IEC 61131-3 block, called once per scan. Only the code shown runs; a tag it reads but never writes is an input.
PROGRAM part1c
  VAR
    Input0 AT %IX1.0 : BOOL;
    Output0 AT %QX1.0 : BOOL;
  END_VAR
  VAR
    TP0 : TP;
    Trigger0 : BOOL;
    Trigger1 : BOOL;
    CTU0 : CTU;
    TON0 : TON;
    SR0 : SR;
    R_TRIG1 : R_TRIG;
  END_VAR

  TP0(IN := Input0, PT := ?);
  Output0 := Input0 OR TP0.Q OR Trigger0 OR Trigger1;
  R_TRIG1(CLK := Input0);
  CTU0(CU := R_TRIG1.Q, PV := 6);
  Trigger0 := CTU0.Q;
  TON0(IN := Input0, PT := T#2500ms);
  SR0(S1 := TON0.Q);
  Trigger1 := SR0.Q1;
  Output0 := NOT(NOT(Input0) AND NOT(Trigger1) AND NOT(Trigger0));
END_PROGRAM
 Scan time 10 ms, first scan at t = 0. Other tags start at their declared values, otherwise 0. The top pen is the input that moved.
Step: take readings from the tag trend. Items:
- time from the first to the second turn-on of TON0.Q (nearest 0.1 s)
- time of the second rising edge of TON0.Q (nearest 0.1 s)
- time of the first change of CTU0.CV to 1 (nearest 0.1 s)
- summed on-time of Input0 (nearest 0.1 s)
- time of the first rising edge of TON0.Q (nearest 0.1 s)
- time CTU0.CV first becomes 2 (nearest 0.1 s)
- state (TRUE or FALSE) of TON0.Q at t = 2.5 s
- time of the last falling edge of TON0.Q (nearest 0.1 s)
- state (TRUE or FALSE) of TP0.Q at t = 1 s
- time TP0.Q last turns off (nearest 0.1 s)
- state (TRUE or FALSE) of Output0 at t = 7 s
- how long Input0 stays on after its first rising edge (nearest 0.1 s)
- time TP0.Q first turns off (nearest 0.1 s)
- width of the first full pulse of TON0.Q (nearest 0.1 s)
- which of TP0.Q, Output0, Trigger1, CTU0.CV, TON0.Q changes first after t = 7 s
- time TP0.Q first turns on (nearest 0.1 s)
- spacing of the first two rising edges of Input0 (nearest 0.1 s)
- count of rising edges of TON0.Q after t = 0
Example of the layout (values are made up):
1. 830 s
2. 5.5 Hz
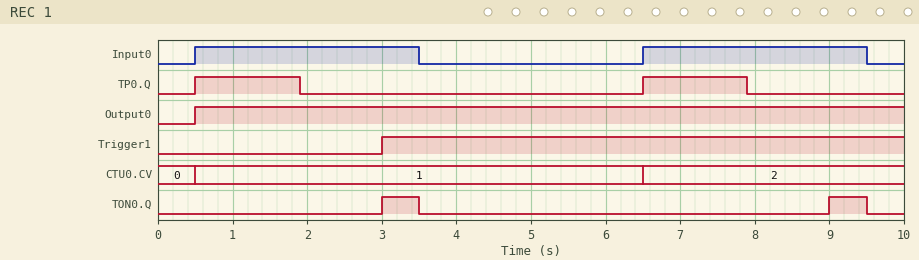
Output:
1. 6.0 s
2. 9.0 s
3. 0.5 s
4. 6.0 s
5. 3.0 s
6. 6.5 s
7. FALSE
8. 9.5 s
9. TRUE
10. 7.9 s
11. TRUE
12. 3.0 s
13. 1.9 s
14. 0.5 s
15. TP0.Q
16. 0.5 s
17. 6.0 s
18. 2
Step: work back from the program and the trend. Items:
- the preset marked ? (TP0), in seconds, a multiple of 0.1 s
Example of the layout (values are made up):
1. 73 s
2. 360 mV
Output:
1. 1.4 s
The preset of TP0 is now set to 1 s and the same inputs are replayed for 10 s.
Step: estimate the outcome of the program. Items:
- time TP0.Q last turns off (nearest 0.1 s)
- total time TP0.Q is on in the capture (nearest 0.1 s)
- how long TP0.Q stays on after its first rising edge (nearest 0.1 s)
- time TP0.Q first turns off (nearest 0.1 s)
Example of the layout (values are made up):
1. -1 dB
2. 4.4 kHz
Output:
1. 7.5 s
2. 2.0 s
3. 1.0 s
4. 1.5 s
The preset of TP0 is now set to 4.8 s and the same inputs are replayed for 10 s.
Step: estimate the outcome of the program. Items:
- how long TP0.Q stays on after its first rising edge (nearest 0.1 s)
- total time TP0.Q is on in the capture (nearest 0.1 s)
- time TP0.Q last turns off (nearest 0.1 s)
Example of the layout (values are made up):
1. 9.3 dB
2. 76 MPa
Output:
1. 4.8 s
2. 8.3 s
3. 5.3 s
